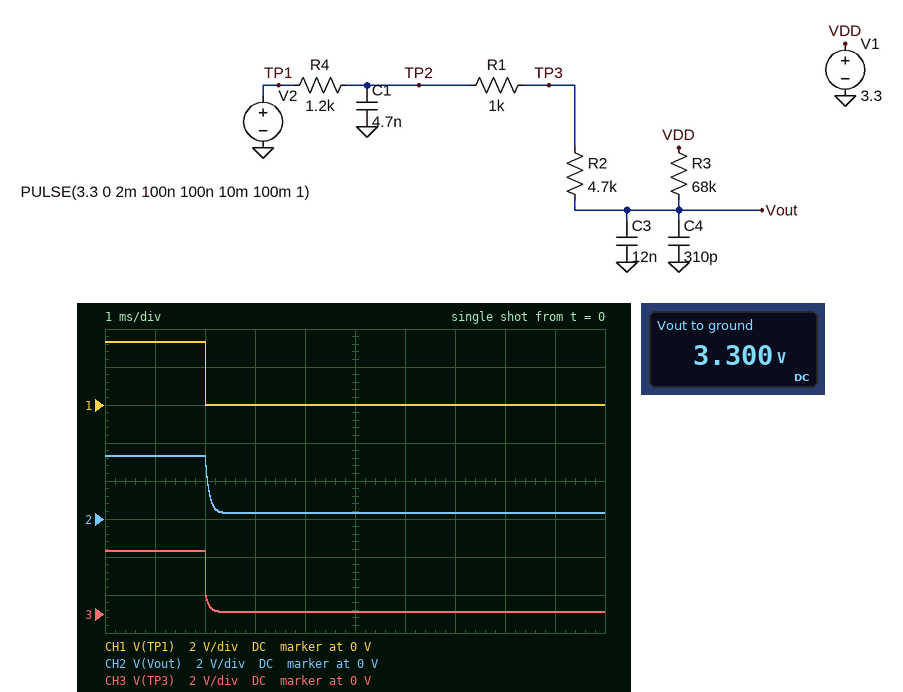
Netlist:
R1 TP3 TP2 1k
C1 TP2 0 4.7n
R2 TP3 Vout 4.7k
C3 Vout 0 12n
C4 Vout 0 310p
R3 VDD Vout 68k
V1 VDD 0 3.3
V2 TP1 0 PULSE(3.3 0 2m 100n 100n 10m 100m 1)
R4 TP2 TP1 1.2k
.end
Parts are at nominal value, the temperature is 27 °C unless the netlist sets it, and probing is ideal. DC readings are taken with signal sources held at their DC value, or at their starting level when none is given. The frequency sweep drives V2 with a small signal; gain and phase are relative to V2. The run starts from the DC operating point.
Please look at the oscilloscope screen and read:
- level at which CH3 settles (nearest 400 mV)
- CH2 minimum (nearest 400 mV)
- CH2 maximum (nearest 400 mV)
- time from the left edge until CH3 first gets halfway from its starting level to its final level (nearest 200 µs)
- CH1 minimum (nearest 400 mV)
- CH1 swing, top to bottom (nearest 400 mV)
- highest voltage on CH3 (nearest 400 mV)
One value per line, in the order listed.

0 V
400 mV
3.2 V
2.0 ms
0 V
3.2 V
3.2 V
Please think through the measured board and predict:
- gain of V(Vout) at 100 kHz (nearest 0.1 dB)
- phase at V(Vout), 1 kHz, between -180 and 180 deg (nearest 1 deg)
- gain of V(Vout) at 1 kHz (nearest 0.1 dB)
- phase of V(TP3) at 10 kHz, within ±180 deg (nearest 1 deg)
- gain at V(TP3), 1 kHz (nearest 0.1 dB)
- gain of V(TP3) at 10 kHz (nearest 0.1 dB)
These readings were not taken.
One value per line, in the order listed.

-44.4 dB
-28 deg
-1.8 dB
-21 deg
-0.7 dB
-3.6 dB
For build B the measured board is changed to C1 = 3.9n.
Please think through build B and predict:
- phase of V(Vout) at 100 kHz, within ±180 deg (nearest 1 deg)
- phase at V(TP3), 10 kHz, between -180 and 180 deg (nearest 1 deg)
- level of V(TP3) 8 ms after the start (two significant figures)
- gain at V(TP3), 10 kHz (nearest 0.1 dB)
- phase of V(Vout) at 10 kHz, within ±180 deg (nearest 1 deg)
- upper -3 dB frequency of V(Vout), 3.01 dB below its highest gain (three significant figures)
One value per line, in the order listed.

-156 deg
-18 deg
97 mV
-3.5 dB
-92 deg
2.04 kHz
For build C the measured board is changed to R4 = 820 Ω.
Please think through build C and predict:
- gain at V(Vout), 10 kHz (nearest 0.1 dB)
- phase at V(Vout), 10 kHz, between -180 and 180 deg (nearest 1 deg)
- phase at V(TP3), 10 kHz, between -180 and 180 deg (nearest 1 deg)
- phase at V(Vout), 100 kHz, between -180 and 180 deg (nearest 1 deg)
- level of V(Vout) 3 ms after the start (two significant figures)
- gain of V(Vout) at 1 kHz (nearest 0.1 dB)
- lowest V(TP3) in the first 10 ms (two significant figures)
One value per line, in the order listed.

-14.5 dB
-90 deg
-16 deg
-153 deg
290 mV
-1.6 dB
81 mV
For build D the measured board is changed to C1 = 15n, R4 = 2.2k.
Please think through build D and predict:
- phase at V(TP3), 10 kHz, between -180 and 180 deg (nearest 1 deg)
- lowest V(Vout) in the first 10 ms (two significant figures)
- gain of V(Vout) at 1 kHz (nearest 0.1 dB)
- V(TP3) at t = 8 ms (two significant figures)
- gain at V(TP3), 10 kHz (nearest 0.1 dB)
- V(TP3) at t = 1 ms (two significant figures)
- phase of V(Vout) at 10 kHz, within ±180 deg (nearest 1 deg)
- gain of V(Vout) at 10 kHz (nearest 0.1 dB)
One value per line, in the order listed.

-60 deg
340 mV
-2.4 dB
140 mV
-9.7 dB
3.3 V
-134 deg
-21.3 dB
